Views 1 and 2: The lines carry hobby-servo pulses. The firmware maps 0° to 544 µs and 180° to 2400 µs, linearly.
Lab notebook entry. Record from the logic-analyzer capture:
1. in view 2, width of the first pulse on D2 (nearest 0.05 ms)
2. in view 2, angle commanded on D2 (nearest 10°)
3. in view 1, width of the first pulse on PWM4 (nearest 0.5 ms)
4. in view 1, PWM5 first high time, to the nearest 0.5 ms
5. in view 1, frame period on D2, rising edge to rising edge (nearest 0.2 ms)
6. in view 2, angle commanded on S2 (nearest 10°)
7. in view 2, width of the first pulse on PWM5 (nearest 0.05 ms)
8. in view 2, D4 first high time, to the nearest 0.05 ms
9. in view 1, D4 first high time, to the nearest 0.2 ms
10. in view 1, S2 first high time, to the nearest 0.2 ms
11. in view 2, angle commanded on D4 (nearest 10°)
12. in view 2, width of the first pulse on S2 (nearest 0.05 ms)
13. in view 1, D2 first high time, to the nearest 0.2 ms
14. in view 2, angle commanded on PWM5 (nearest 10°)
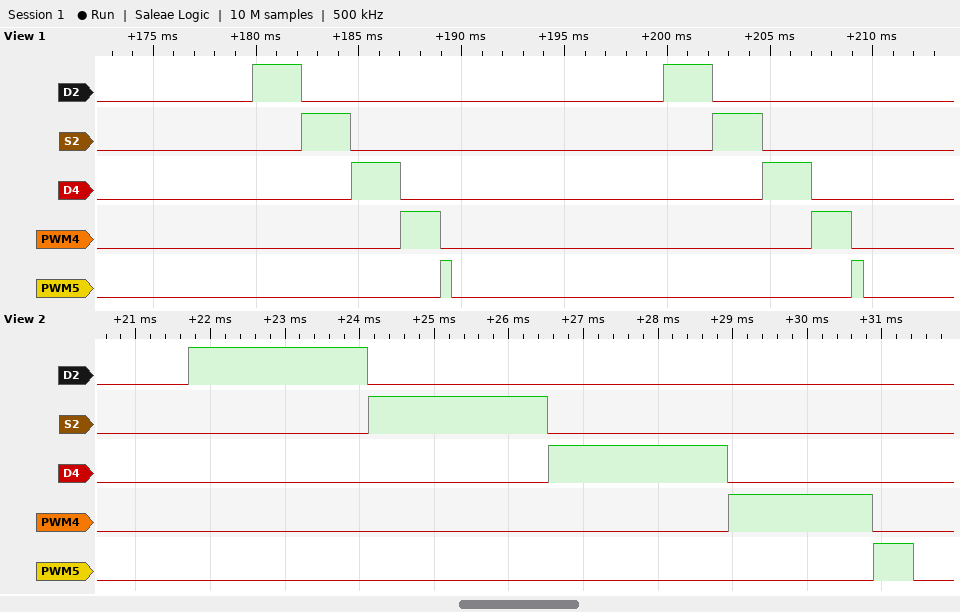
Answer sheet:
2.40 ms
180°
2.0 ms
0.5 ms
20.0 ms
180°
0.55 ms
2.40 ms
2.4 ms
2.4 ms
180°
2.40 ms
2.4 ms
0°
